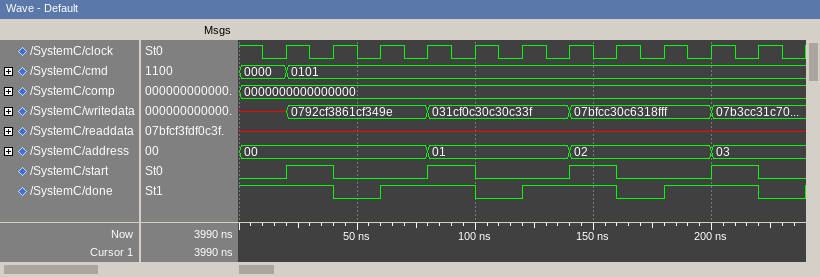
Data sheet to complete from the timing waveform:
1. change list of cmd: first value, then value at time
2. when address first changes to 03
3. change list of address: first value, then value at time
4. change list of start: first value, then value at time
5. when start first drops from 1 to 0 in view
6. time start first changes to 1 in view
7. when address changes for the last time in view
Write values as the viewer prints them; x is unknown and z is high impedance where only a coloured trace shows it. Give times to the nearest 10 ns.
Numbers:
0000, 0101 at 20 ns
200 ns
00, 01 at 80 ns, 02 at 140 ns, 03 at 200 ns
0, 1 at 20 ns, 0 at 40 ns, 1 at 80 ns, 0 at 100 ns, 1 at 140 ns, 0 at 160 ns, 1 at 200 ns, 0 at 220 ns
40 ns
20 ns
200 ns
